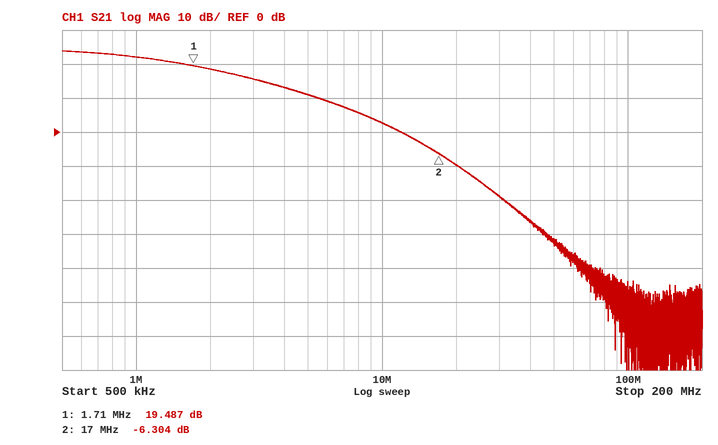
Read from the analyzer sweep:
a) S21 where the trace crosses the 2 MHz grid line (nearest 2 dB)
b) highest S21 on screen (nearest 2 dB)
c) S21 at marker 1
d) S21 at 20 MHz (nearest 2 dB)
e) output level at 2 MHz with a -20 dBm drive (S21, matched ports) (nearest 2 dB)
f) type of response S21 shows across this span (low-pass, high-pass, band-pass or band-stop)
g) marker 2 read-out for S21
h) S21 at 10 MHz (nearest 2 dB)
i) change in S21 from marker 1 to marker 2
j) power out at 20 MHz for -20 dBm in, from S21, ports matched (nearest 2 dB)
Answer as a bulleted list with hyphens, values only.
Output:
- 18 dB
- 24 dB
- 19.487 dB
- -10 dB
- -2 dBm
- low-pass
- -6.304 dB
- 2 dB
- -25.791 dB
- -30 dBm
